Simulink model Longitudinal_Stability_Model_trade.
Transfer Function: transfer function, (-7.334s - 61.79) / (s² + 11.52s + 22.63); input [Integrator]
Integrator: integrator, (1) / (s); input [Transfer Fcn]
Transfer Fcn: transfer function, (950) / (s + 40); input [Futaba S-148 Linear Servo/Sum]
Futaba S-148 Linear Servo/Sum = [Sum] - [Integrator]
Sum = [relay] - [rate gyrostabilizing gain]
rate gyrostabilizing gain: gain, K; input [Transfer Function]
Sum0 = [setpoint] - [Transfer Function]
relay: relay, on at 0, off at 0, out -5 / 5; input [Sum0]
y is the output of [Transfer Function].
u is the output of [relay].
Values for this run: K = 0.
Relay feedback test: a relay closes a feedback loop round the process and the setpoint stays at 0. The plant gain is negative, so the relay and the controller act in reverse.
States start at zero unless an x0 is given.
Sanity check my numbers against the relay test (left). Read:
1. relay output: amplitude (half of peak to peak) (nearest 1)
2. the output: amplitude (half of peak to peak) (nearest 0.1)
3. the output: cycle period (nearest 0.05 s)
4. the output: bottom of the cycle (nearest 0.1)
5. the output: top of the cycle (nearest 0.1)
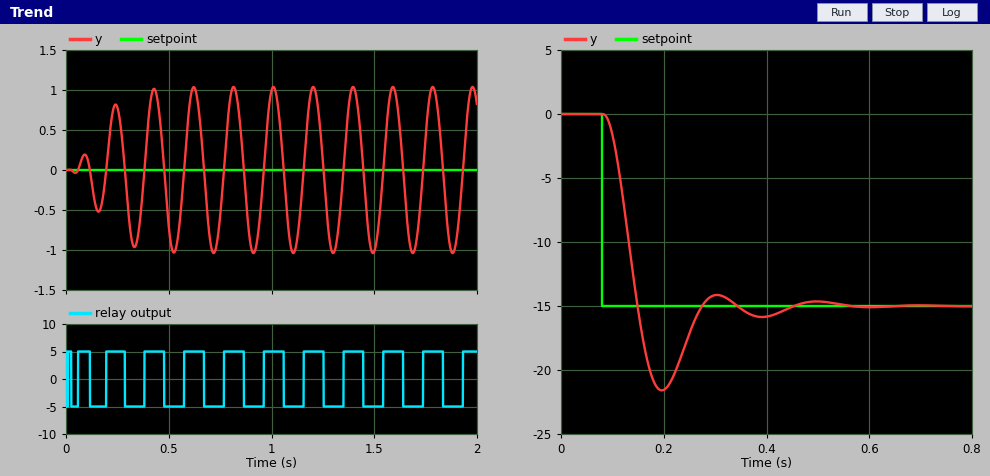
5
1.0
0.20 s
-1.0
1.0
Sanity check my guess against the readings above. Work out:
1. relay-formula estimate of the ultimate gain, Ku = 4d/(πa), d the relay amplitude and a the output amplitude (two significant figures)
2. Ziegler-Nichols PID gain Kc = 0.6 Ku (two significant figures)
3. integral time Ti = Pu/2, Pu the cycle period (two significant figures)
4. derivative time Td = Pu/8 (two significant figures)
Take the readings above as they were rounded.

6.4
3.8
0.10 s
0.025 s
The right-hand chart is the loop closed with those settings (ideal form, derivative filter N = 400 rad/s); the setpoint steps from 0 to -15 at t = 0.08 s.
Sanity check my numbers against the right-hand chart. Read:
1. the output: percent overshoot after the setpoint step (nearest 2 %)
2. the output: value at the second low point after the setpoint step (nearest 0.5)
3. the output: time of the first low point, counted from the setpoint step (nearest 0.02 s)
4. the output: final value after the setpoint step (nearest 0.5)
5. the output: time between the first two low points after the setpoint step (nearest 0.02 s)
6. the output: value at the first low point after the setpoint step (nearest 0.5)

44 %
-16.0
0.12 s
-15.0
0.20 s
-21.5
